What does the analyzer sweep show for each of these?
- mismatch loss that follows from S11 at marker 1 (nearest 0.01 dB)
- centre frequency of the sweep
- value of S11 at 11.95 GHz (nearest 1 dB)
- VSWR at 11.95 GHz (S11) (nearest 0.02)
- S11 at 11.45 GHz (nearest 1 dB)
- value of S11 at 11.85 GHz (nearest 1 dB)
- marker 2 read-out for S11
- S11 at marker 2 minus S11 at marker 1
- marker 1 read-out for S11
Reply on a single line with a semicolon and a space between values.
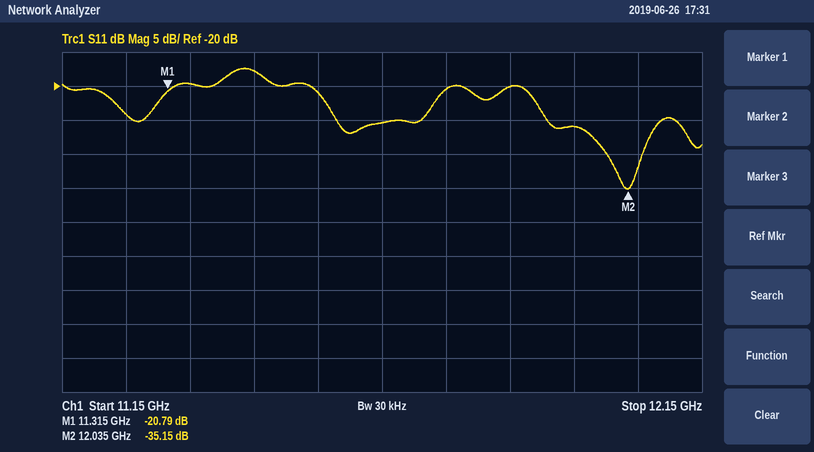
0.04 dB; 11.65 GHz; -26 dB; 1.10; -18 dB; -20 dB; -35.15 dB; -14.36 dB; -20.79 dB
